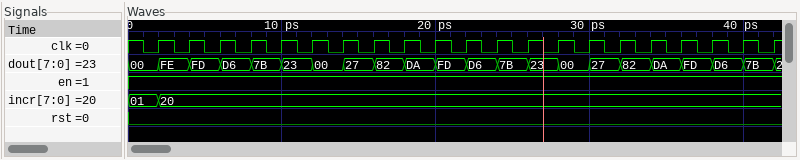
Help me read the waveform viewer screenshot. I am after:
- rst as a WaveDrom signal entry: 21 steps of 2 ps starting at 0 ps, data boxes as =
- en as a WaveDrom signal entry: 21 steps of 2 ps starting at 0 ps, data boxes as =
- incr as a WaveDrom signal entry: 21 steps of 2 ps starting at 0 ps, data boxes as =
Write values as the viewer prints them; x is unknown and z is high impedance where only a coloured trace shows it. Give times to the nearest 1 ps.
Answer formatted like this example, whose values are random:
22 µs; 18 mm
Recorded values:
{name: 'rst', wave: '0....................'}; {name: 'en', wave: '1....................'}; {name: 'incr', wave: '==...................', data: '01 20'}
